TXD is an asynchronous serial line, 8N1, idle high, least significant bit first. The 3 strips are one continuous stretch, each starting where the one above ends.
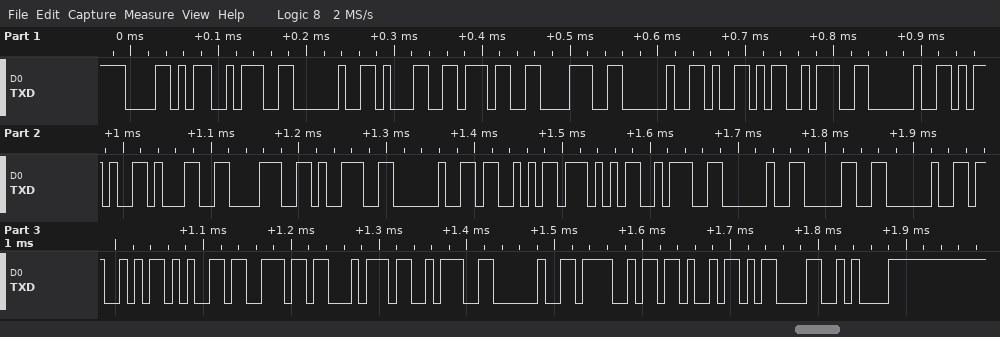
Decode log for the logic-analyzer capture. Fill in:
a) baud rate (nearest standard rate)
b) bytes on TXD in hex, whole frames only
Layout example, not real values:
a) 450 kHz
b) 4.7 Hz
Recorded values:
a) 115200 baud
b) 58 3A 20 31 37 38 20 59 3A 20 2D 31 38 39 20 53 57 3A 20 30 20 53 65 6E 74 3A 20 4F 4B 0D 0A
